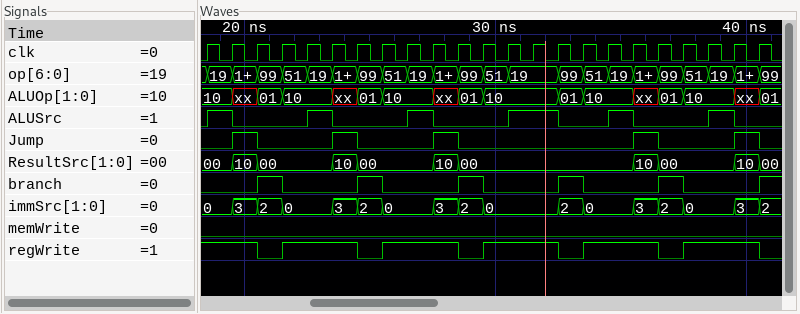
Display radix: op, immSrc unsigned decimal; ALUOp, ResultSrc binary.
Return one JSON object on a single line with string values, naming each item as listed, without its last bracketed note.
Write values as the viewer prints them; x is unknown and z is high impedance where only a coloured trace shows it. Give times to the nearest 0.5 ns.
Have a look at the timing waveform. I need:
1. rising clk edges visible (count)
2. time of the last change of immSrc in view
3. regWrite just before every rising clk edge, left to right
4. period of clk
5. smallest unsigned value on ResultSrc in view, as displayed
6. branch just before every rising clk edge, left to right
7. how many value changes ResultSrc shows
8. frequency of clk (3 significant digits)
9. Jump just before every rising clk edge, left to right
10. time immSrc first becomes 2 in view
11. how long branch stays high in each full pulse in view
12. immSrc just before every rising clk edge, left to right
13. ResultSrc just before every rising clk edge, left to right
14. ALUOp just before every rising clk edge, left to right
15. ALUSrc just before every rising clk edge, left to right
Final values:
{"rising clk edges visible": "23", "time of the last change of immSrc in view": "40.5 ns", "regWrite just before every rising clk edge, left to right": "1 1 1 0 1 1 1 0 1 1 1 0 1 1 1 0 1 1 1 0 1 1 1", "period of clk": "1 ns", "smallest unsigned value on ResultSrc in view, as displayed": "00", "branch just before every rising clk edge, left to right": "0 0 0 1 0 0 0 1 0 0 0 1 0 0 0 1 0 0 0 1 0 0 0", "how many value changes ResultSrc shows": "10", "frequency of clk": "1.00 GHz", "Jump just before every rising clk edge, left to right": "0 0 1 0 0 0 1 0 0 0 1 0 0 0 0 0 0 0 1 0 0 0 1", "time immSrc first becomes 2 in view": "20.5 ns", "how long branch stays high in each full pulse in view": "1 ns, 1 ns, 1 ns, 1 ns, 1 ns", "immSrc just before every rising clk edge, left to right": "0, 0, 3, 2, 0, 0, 3, 2, 0, 0, 3, 2, 0, 0, 0, 2, 0, 0, 3, 2, 0, 0, 3", "ResultSrc just before every rising clk edge, left to right": "00, 00, 10, 00, 00, 00, 10, 00, 00, 00, 10, 00, 00, 00, 00, 00, 00, 00, 10, 00, 00, 00, 10", "ALUOp just before every rising clk edge, left to right": "10, 10, xx, 01, 10, 10, xx, 01, 10, 10, xx, 01, 10, 10, 10, 01, 10, 10, xx, 01, 10, 10, xx", "ALUSrc just before every rising clk edge, left to right": "0 1 0 0 0 1 0 0 0 1 0 0 0 1 1 0 0 1 0 0 0 1 0"}
